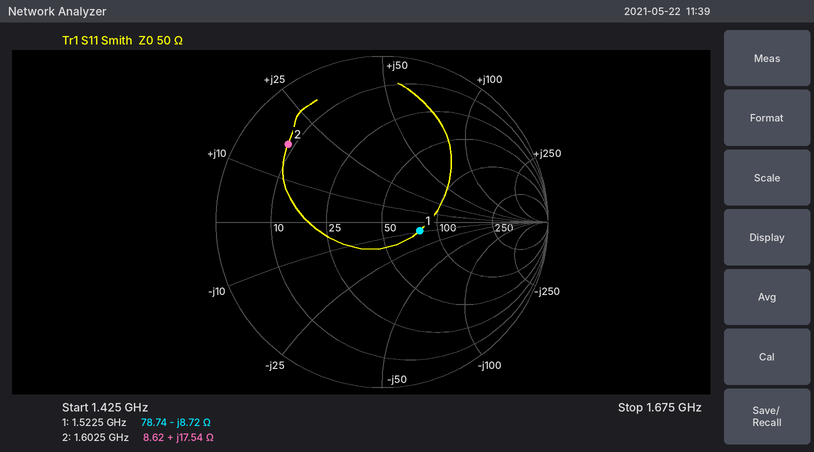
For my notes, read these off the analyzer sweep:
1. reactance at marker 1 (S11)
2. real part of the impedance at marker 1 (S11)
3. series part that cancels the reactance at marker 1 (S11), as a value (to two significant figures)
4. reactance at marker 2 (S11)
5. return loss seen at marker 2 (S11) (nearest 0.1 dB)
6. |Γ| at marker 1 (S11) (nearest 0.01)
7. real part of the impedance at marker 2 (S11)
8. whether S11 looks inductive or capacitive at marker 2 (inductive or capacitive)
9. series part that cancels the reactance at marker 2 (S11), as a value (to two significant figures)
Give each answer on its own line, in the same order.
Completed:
-8.72 Ω
78.74 Ω
910 pH
+17.54 Ω
2.7 dB
0.23
8.62 Ω
inductive
5.7 pF
